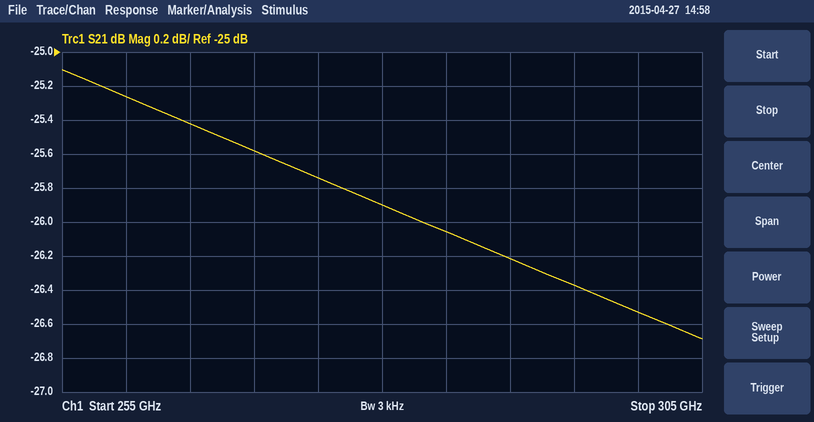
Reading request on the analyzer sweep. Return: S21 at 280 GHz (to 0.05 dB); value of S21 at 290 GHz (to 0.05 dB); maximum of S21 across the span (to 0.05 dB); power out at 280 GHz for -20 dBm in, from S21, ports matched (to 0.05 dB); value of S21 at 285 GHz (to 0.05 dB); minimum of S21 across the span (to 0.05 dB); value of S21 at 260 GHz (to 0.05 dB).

-25.90 dB
-26.20 dB
-25.10 dB
-45.90 dBm
-26.05 dB
-26.70 dB
-25.25 dB
